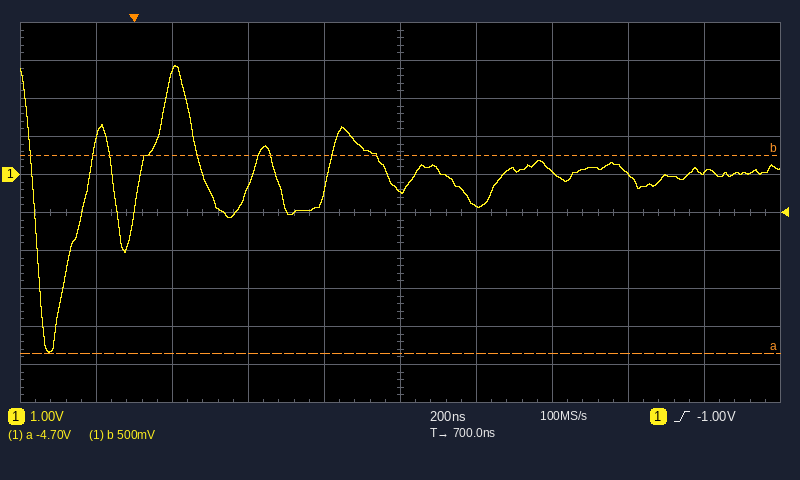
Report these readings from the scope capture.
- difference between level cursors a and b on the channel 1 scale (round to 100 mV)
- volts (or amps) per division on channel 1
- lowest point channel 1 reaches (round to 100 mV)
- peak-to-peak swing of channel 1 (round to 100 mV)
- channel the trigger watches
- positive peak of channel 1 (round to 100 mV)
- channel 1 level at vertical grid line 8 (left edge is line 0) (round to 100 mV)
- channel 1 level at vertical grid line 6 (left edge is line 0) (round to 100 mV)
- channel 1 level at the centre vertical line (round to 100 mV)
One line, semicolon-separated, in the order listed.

5.2 V; 1 V; -4.7 V; 7.6 V; channel 1; 2.9 V; 0.0 V; -800 mV; -400 mV
